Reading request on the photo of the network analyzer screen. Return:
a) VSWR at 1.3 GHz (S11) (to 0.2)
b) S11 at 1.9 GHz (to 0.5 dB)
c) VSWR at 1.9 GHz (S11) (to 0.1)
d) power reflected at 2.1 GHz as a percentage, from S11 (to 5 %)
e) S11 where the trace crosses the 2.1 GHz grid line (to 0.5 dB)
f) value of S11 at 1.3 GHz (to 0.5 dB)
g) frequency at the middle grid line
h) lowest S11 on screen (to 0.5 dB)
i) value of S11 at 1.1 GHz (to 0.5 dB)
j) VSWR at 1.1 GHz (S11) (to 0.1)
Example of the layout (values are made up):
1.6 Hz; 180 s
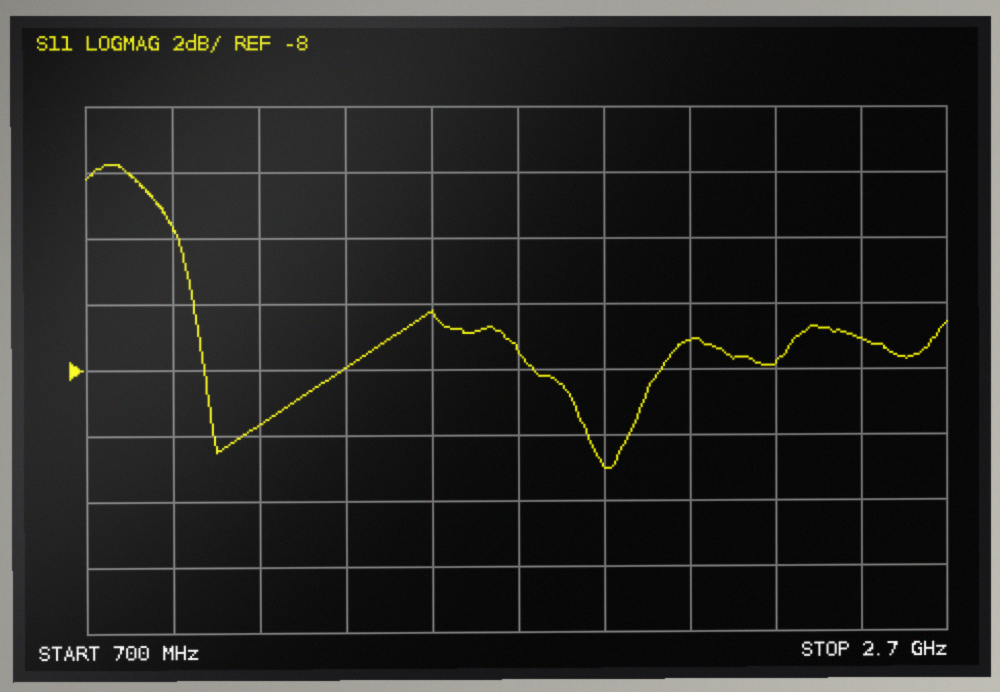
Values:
2.4; -11.0 dB; 1.8; 20 %; -7.0 dB; -8.0 dB; 1.7 GHz; -11.0 dB; -9.5 dB; 2.0
